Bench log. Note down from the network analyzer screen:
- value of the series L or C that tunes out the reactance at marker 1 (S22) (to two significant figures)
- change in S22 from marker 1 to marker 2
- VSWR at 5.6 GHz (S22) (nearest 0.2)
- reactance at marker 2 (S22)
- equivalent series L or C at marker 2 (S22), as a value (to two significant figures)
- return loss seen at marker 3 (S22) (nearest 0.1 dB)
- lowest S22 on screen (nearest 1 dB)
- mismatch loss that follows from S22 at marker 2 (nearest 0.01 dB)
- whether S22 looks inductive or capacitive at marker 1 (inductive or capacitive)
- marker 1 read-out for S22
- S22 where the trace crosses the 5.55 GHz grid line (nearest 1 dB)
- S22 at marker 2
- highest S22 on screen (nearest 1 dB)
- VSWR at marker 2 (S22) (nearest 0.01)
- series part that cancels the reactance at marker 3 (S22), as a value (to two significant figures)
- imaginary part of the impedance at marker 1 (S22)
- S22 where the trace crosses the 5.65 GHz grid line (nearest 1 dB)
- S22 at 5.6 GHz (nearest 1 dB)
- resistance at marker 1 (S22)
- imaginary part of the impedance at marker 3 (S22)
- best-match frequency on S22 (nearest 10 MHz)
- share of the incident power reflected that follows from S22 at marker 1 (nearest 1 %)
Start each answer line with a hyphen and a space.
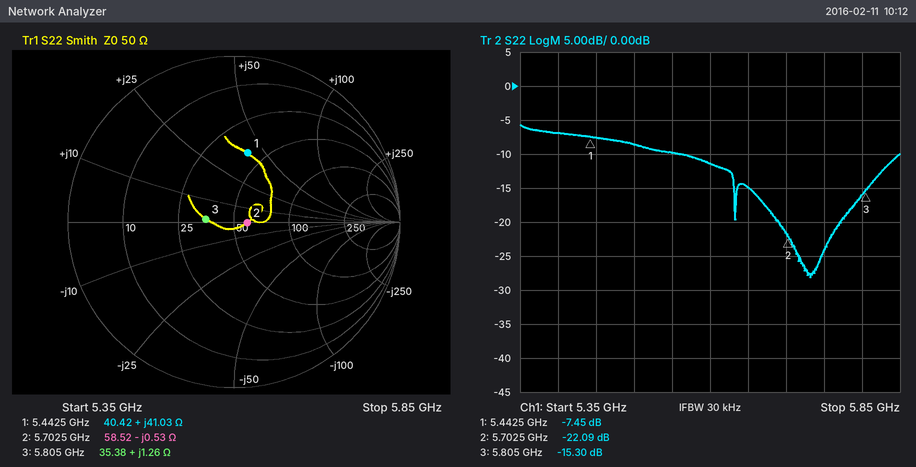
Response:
- 710 fF
- -14.64 dB
- 1.8
- -0.53 Ω
- 53 pF
- 15.3 dB
- -28 dB
- 0.03 dB
- inductive
- -7.45 dB
- -10 dB
- -22.09 dB
- -6 dB
- 1.17
- 22 pF
- +41.03 Ω
- -15 dB
- -11 dB
- 40.42 Ω
- +1.26 Ω
- 5.73 GHz
- 18 %
